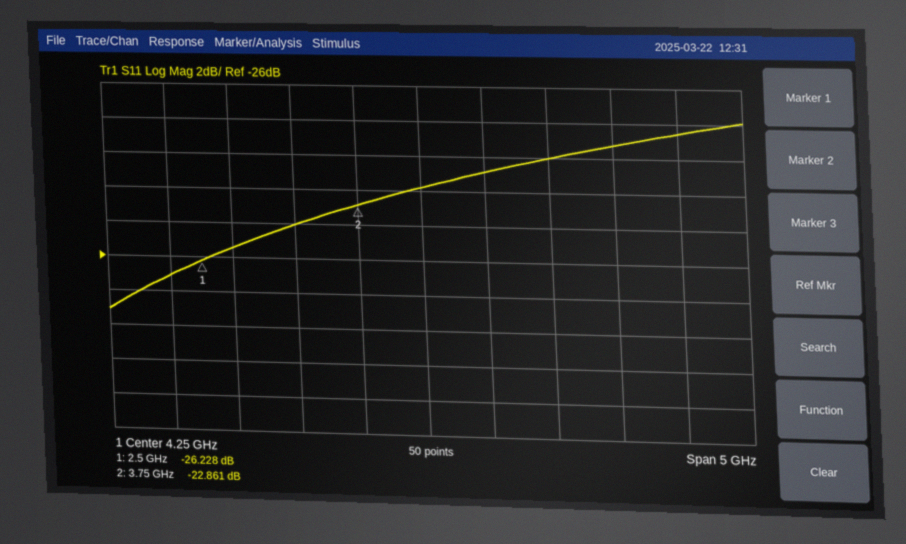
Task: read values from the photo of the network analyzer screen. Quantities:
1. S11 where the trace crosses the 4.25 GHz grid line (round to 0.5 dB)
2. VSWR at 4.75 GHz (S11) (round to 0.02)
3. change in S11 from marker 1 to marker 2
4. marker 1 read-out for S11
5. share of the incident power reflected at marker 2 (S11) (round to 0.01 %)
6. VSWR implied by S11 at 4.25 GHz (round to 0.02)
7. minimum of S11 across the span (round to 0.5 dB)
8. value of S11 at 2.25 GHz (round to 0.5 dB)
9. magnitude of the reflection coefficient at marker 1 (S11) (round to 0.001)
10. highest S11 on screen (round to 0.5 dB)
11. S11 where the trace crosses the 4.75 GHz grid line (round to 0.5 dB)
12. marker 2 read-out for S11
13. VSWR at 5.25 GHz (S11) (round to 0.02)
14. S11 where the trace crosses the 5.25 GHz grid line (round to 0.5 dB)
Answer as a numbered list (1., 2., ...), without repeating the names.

1. -22.0 dB
2. 1.20
3. 3.367 dB
4. -26.228 dB
5. 0.52 %
6. 1.18
7. -29.0 dB
8. -27.0 dB
9. 0.049
10. -18.0 dB
11. -21.0 dB
12. -22.861 dB
13. 1.22
14. -20.0 dB
